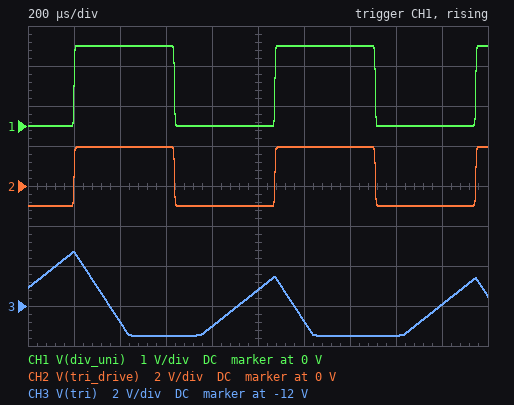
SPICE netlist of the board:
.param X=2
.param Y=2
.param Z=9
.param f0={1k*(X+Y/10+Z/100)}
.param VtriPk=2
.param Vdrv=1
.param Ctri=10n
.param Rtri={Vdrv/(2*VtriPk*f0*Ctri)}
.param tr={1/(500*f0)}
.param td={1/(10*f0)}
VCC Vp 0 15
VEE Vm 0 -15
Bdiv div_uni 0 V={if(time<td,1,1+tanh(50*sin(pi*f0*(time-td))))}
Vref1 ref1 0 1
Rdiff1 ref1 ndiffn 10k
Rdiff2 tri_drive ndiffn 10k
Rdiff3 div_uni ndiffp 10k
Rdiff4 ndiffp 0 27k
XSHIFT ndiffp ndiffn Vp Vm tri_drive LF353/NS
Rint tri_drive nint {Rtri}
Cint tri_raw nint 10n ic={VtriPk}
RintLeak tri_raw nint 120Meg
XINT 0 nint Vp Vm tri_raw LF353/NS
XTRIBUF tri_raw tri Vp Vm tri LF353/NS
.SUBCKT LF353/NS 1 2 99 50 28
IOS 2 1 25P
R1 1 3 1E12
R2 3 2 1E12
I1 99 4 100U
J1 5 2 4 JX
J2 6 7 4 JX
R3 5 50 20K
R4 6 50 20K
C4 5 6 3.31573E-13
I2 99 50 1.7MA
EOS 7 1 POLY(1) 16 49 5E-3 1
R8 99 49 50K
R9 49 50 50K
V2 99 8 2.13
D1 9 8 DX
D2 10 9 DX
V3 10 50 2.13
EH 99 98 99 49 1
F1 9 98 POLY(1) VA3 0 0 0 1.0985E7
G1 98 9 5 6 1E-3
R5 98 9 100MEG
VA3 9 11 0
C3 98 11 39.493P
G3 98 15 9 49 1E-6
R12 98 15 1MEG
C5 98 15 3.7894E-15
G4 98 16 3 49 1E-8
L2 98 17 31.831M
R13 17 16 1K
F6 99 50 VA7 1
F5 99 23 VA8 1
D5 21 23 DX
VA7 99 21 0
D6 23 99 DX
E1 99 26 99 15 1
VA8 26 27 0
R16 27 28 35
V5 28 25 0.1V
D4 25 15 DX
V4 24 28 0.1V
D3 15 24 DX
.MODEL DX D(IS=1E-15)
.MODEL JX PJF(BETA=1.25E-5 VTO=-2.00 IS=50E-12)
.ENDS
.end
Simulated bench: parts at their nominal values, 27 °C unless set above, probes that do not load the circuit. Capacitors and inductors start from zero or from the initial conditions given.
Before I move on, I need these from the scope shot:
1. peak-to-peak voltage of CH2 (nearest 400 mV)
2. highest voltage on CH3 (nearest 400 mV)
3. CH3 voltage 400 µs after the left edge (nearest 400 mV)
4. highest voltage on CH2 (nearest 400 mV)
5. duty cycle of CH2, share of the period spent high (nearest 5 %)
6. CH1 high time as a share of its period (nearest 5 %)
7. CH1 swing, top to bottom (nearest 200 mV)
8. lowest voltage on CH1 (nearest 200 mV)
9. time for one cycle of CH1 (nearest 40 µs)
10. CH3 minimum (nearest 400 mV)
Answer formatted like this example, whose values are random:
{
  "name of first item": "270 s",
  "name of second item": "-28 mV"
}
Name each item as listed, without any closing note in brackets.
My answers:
{
  "peak-to-peak voltage of CH2": "2.8 V",
  "highest voltage on CH3": "-9.2 V",
  "CH3 voltage 400 µs after the left edge": "-12.8 V",
  "highest voltage on CH2": "2.0 V",
  "duty cycle of CH2, share of the period spent high": "50 %",
  "CH1 high time as a share of its period": "50 %",
  "CH1 swing, top to bottom": "2.0 V",
  "lowest voltage on CH1": "0 V",
  "time for one cycle of CH1": "880 µs",
  "CH3 minimum": "-13.6 V"
}
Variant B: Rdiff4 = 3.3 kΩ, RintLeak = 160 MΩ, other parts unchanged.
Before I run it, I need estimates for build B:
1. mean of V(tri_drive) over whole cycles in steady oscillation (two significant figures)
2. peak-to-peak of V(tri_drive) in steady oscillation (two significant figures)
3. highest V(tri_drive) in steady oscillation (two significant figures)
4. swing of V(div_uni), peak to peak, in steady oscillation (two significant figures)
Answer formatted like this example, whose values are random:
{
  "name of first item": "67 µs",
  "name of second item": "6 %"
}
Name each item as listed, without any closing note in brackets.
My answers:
{
  "mean of V(tri_drive) over whole cycles in steady oscillation": "-490 mV",
  "peak-to-peak of V(tri_drive) in steady oscillation": "990 mV",
  "highest V(tri_drive) in steady oscillation": "2.5 mV",
  "swing of V(div_uni), peak to peak, in steady oscillation": "2.0 V"
}
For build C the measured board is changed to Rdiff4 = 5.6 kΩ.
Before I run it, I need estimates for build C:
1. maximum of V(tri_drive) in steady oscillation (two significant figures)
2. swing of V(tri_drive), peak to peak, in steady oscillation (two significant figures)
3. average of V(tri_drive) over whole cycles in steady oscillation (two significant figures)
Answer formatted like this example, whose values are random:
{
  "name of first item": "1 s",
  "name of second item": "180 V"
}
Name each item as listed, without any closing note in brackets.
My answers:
{
  "maximum of V(tri_drive) in steady oscillation": "450 mV",
  "swing of V(tri_drive), peak to peak, in steady oscillation": "1.4 V",
  "average of V(tri_drive) over whole cycles in steady oscillation": "-270 mV"
}
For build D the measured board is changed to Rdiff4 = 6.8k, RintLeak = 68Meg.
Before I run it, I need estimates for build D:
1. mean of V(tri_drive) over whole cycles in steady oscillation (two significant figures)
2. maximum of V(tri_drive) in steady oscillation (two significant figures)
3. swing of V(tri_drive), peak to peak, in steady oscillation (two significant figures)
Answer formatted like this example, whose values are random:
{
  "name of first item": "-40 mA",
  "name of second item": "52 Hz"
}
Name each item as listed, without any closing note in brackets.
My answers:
{
  "mean of V(tri_drive) over whole cycles in steady oscillation": "-180 mV",
  "maximum of V(tri_drive) in steady oscillation": "630 mV",
  "swing of V(tri_drive), peak to peak, in steady oscillation": "1.6 V"
}
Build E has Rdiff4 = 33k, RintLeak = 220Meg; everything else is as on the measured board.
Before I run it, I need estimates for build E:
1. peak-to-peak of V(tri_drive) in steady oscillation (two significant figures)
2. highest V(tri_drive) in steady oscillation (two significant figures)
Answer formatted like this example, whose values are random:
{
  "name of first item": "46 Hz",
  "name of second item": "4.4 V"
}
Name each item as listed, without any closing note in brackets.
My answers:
{
  "peak-to-peak of V(tri_drive) in steady oscillation": "3.1 V",
  "highest V(tri_drive) in steady oscillation": "2.1 V"
}
